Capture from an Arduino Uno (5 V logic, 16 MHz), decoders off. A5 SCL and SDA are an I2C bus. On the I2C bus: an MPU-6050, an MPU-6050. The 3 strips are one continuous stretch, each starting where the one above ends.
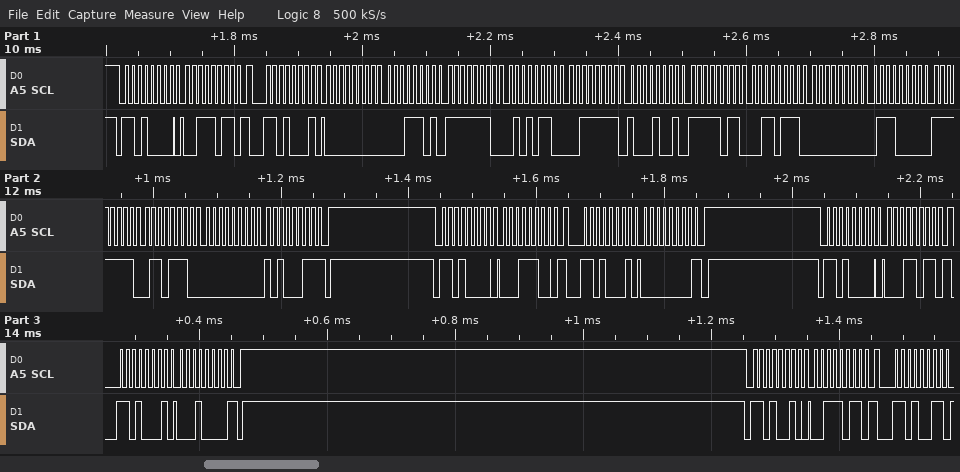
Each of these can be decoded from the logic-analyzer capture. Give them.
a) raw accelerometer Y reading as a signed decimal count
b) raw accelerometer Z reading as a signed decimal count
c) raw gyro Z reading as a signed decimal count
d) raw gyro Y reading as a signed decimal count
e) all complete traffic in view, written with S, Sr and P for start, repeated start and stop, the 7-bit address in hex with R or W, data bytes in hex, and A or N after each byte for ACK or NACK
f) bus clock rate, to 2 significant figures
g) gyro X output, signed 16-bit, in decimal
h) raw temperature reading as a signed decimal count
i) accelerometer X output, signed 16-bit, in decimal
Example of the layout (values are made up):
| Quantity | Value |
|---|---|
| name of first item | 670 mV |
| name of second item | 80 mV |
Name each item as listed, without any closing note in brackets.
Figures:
| Quantity | Value |
|---|---|
| raw accelerometer Y reading as a signed decimal count | -426 |
| raw accelerometer Z reading as a signed decimal count | 16265 |
| raw gyro Z reading as a signed decimal count | 163 |
| raw gyro Y reading as a signed decimal count | -146 |
| all complete traffic in view, written with S, Sr and P for start, repeated start and stop, the 7-bit address in hex with R or W, data bytes in hex, and A or N after each byte for ACK or NACK | S 68W A 3B A Sr 68R A 00 A 1D A FE A 56 A 3F A 89 A FB A 37 A 00 A 70 A FF A 6E A 00 A A3 N P S 68W A 1C A Sr 68R A 00 N P S 68W A 1B A Sr 68R A 10 N P S 69W A 3B A Sr 69R A |
| bus clock rate, to 2 significant figures | 100 kHz |
| gyro X output, signed 16-bit, in decimal | 112 |
| raw temperature reading as a signed decimal count | -1225 |
| accelerometer X output, signed 16-bit, in decimal | 29 |
